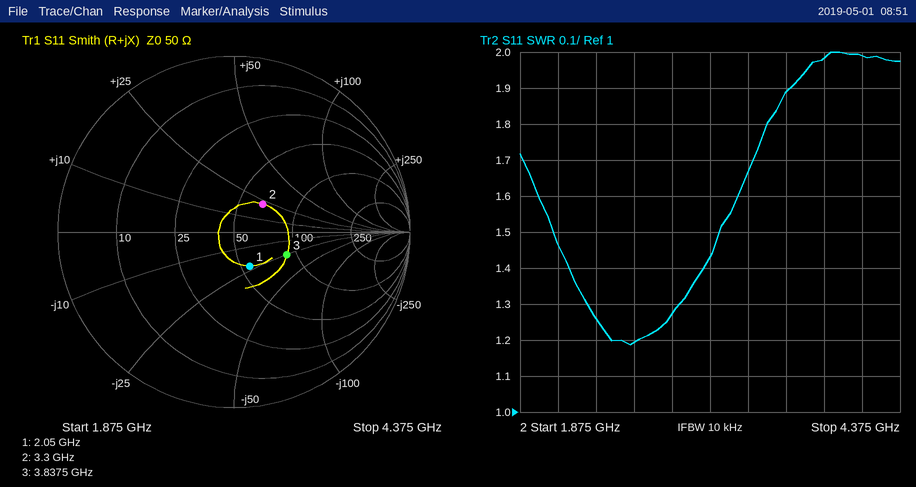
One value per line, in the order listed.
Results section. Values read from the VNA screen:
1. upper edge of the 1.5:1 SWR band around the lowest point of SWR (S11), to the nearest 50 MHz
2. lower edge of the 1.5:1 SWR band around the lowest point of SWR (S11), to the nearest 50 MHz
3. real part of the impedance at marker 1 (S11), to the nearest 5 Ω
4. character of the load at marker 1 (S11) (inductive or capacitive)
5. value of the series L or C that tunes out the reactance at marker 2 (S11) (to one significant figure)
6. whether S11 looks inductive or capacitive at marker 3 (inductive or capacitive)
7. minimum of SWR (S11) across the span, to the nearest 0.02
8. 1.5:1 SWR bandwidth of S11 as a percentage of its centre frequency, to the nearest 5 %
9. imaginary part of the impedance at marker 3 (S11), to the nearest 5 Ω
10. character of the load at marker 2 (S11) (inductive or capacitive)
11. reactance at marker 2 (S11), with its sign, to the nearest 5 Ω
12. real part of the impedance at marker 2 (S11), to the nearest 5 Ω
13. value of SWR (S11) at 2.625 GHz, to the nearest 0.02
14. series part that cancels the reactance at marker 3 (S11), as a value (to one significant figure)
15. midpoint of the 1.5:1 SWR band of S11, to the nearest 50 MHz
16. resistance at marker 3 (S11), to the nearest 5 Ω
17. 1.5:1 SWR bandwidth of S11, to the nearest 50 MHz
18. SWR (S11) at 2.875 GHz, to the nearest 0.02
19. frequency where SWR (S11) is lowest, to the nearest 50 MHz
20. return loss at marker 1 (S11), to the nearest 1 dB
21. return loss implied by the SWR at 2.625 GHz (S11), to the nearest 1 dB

3.20 GHz
2.10 GHz
55 Ω
capacitive
2 pF
capacitive
1.18
40 %
-25 Ω
inductive
+20 Ω
65 Ω
1.20
1 nH
2.65 GHz
90 Ω
1.10 GHz
1.28
2.60 GHz
13 dB
21 dB
